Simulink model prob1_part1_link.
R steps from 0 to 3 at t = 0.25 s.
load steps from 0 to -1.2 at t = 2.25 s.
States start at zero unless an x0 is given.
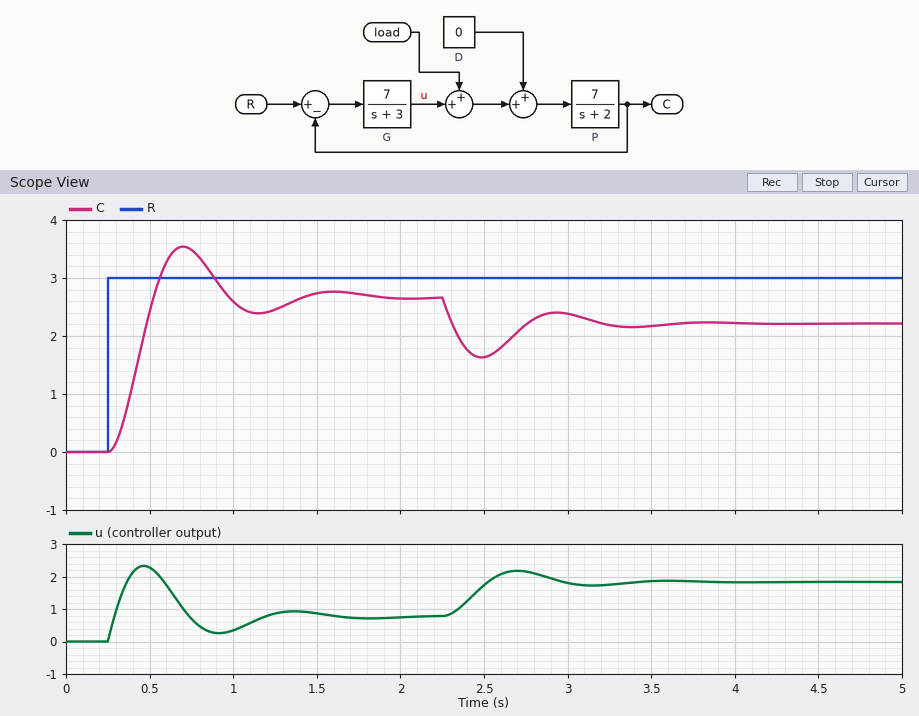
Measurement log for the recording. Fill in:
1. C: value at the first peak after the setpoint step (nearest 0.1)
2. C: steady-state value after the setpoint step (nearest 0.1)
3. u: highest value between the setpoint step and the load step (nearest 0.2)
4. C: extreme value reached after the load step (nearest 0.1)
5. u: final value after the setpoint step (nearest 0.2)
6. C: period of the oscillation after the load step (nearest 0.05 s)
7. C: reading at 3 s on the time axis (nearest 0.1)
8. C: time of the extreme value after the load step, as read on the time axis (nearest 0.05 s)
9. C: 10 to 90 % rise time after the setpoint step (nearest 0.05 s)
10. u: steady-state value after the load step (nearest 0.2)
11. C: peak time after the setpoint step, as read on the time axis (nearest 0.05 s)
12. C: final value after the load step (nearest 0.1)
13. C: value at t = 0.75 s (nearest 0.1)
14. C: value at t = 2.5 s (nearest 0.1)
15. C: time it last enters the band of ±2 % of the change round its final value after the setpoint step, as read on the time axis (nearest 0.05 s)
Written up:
3.5
2.7
2.4
1.6
0.8
0.90 s
2.4
2.50 s
0.20 s
1.8
0.70 s
2.2
3.5
1.6
1.75 s
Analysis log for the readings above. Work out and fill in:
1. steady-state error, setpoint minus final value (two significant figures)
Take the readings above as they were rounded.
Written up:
0.30
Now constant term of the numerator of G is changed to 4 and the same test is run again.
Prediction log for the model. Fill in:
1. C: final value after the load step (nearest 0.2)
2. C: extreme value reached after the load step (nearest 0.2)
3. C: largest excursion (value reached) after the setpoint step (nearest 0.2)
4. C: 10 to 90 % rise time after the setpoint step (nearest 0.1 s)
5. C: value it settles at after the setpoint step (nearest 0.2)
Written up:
1.8
1.2
3.0
0.3 s
2.4
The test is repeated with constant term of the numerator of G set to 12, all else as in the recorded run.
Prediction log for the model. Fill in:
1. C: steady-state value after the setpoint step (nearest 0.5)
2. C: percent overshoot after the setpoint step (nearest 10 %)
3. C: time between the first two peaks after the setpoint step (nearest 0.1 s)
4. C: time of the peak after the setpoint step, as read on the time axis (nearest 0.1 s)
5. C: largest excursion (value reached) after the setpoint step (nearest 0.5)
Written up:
3.0
40 %
0.7 s
0.6 s
4.0
